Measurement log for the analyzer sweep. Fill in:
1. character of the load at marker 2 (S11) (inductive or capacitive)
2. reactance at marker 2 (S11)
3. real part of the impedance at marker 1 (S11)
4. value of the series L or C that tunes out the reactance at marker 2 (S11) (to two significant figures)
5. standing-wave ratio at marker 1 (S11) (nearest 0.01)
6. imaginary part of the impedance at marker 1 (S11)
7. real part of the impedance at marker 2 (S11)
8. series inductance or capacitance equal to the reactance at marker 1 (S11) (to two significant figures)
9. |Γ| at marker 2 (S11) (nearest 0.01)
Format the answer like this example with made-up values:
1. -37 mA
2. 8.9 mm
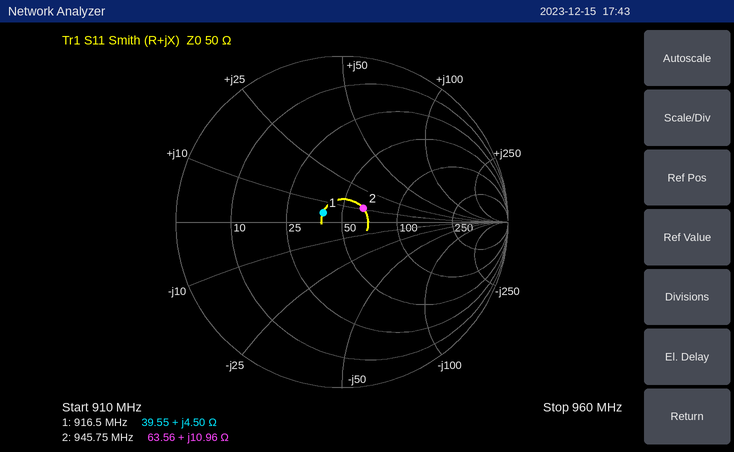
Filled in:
1. inductive
2. +10.96 Ω
3. 39.55 Ω
4. 15 pF
5. 1.29
6. +4.50 Ω
7. 63.56 Ω
8. 780 pH
9. 0.15
